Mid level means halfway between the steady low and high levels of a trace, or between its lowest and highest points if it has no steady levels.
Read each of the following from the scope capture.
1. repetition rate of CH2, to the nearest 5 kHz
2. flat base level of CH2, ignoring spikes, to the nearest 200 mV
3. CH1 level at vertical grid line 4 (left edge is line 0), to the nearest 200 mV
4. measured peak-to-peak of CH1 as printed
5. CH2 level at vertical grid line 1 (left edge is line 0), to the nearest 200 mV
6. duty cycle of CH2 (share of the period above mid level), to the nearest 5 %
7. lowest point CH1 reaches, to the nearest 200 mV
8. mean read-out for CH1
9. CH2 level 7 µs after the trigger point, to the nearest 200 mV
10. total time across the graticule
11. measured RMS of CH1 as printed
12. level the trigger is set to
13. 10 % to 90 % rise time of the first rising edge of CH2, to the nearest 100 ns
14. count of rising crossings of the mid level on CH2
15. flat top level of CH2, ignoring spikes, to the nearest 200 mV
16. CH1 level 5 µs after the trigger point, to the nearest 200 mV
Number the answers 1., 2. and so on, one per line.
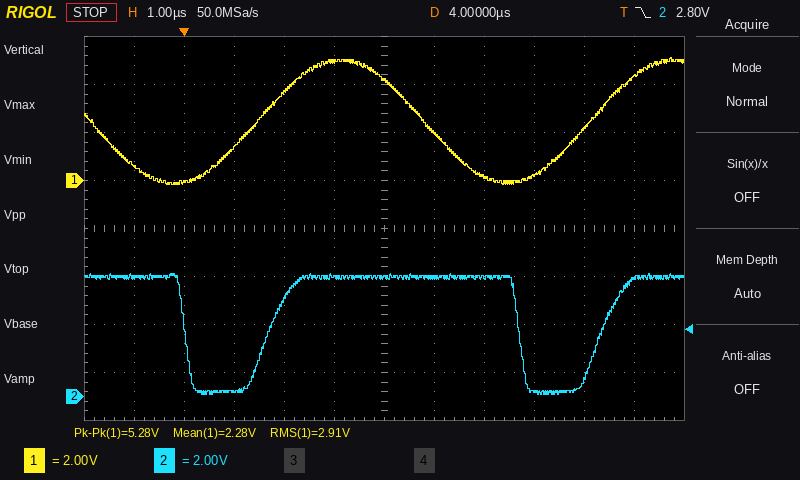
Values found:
1. 150 kHz
2. 200 mV
3. 3.6 V
4. 5.28 V
5. 5.0 V
6. 75 %
7. -200 mV
8. 2.28 V
9. 200 mV
10. 12 µs
11. 2.91 V
12. 2.80 V
13. 800 ns
14. 2
15. 5.0 V
16. 2.0 V
